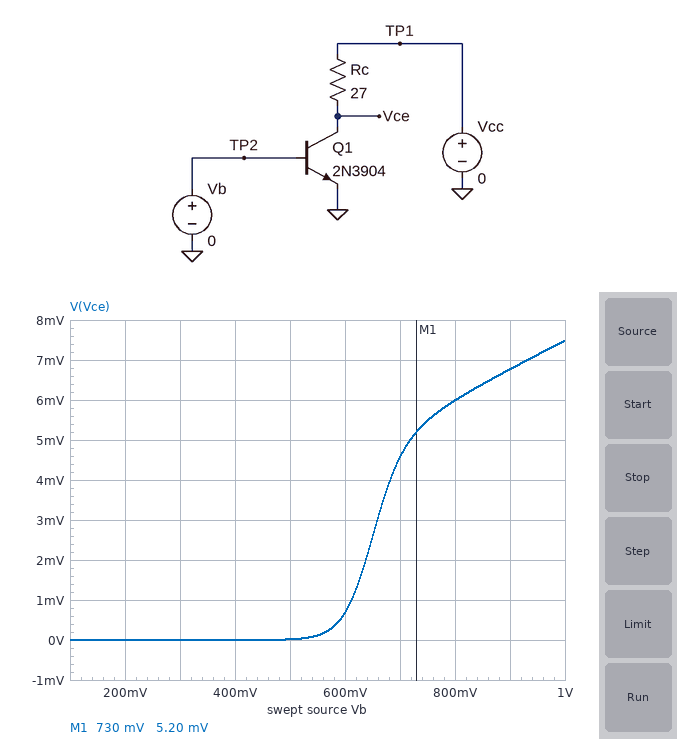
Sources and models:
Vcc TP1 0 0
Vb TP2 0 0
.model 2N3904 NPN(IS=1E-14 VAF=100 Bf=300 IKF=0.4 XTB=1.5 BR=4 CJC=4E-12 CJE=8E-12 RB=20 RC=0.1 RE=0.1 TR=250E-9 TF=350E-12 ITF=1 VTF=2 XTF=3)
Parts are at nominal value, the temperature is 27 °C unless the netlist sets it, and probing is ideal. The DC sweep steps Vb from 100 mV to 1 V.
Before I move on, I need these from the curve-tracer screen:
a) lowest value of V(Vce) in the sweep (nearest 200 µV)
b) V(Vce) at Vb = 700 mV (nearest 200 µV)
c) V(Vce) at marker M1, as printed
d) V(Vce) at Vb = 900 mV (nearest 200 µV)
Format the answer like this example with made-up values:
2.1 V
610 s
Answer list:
0 V
4.6 mV
5.20 mV
6.8 mV
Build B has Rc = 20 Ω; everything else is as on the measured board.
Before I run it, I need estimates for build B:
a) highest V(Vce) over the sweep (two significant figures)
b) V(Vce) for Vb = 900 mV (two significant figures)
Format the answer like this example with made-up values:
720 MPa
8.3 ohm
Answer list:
7.4 mV
6.7 mV
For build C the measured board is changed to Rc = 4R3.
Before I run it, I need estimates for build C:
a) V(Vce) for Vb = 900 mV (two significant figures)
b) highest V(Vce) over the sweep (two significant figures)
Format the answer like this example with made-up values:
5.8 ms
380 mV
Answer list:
5.7 mV
6.6 mV
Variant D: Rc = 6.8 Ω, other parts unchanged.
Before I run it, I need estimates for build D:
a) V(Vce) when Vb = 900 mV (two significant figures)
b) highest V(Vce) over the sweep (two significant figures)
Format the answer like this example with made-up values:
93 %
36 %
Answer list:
6.1 mV
7.0 mV
